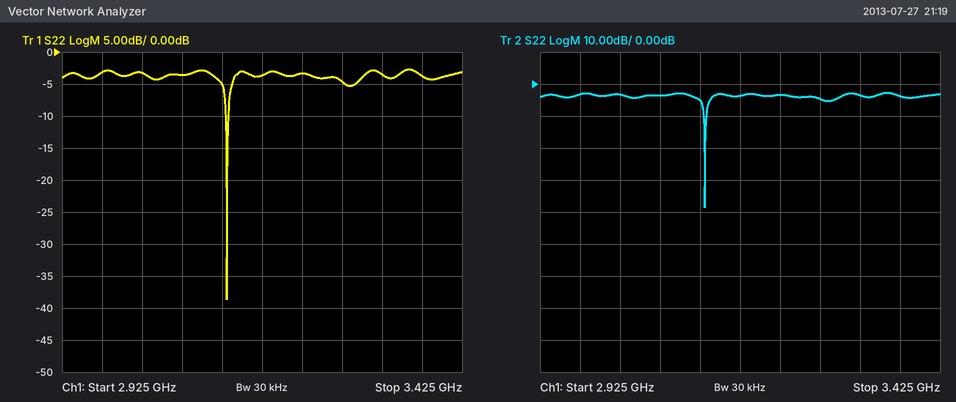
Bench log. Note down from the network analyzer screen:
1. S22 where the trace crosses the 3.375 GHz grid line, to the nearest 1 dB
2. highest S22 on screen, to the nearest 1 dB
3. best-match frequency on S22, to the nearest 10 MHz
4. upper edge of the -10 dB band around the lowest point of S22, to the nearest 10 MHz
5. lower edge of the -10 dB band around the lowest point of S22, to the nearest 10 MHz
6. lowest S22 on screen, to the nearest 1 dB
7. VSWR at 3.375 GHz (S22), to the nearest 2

-4 dB
-3 dB
3.13 GHz
3.13 GHz
3.13 GHz
-39 dB
4
